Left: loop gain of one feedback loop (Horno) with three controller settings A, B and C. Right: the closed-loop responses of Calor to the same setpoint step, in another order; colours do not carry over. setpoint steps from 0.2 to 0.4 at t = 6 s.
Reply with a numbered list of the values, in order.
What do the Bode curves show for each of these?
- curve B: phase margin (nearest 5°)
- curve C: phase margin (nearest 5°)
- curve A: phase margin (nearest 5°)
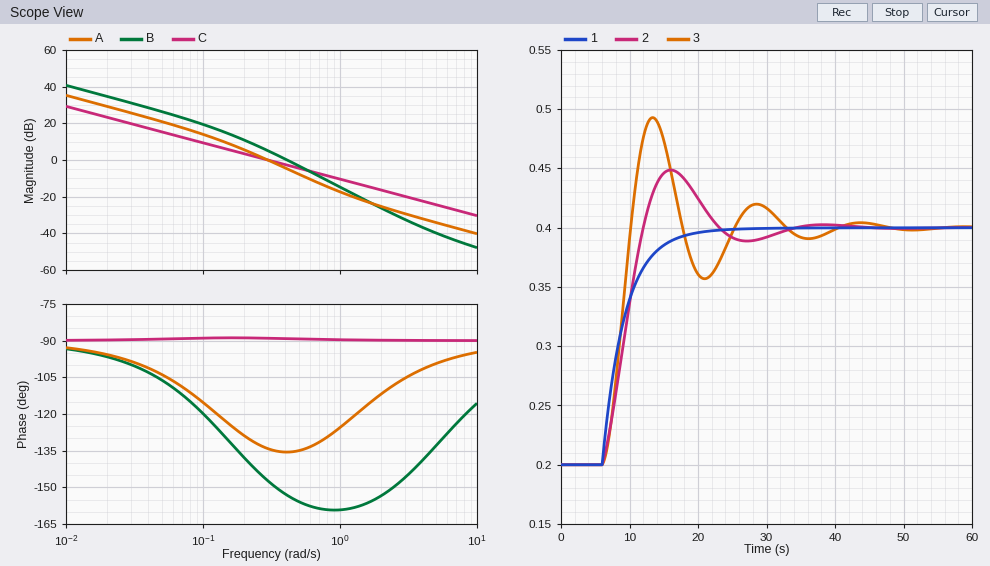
1. 25°
2. 90°
3. 45°
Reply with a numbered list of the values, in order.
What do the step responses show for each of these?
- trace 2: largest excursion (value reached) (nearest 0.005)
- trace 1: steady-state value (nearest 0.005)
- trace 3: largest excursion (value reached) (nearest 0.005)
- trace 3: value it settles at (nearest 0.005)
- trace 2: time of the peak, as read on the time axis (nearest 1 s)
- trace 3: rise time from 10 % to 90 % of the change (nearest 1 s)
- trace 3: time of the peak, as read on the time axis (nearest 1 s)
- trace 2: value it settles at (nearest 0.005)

1. 0.450
2. 0.400
3. 0.495
4. 0.400
5. 16 s
6. 3 s
7. 13 s
8. 0.400
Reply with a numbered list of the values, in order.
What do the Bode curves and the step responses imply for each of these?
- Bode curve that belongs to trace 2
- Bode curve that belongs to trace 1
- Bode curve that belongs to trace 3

1. A
2. C
3. B
